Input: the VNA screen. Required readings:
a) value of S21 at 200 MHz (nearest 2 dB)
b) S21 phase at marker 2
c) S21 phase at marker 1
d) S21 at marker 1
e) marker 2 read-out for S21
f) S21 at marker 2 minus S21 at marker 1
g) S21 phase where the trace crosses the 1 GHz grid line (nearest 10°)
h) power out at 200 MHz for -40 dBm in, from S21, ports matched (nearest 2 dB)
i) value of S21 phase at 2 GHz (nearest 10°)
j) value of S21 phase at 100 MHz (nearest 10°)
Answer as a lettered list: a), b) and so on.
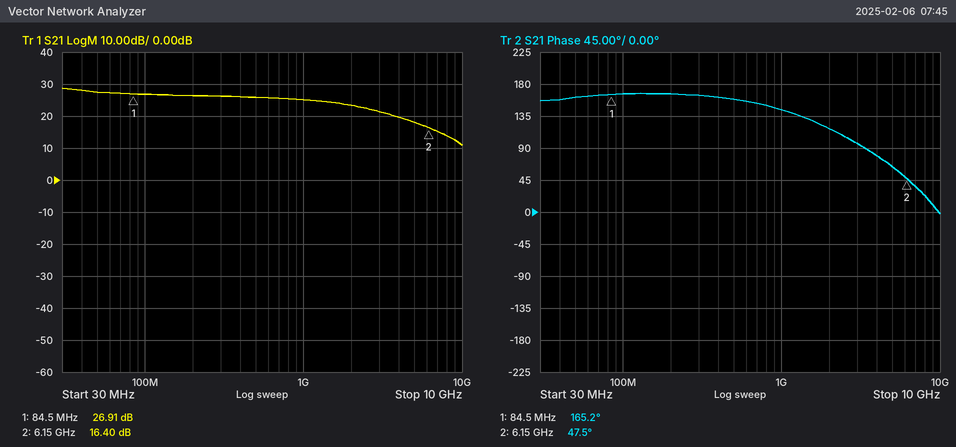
a) 26 dB
b) 47.5°
c) 165.2°
d) 26.91 dB
e) 16.40 dB
f) -10.51 dB
g) 140°
h) -14 dBm
i) 120°
j) 170°
